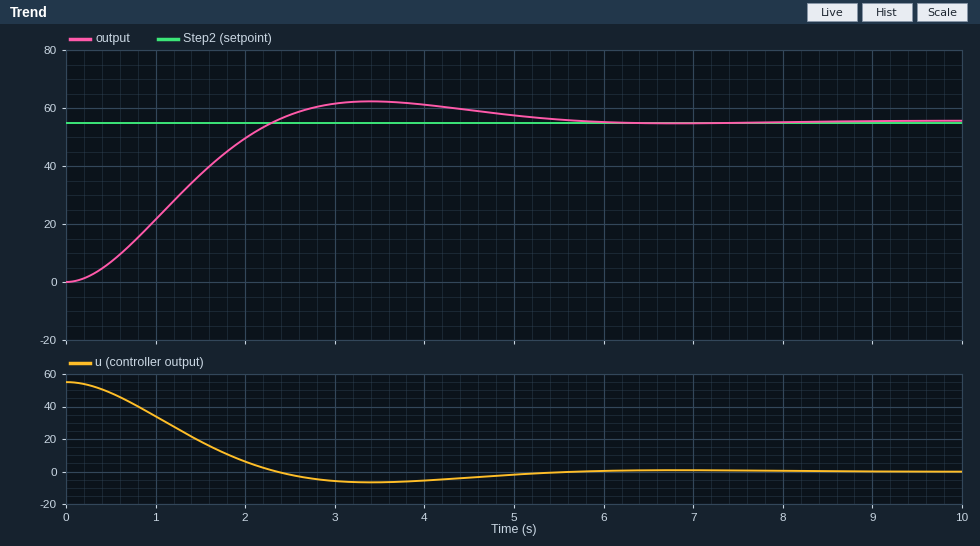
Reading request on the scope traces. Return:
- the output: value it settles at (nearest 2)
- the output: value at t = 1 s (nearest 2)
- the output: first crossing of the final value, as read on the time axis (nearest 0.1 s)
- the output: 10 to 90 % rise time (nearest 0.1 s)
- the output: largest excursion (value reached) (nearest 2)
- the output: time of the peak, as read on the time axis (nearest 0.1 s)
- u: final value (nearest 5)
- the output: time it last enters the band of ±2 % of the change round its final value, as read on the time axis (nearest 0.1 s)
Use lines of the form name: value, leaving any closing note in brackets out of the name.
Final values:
the output: value it settles at: 56
the output: value at t = 1 s: 22
the output: first crossing of the final value, as read on the time axis: 2.3 s
the output: 10 to 90 % rise time: 1.6 s
the output: largest excursion (value reached): 62
the output: time of the peak, as read on the time axis: 3.4 s
u: final value: 0
the output: time it last enters the band of ±2 % of the change round its final value, as read on the time axis: 5.3 s
